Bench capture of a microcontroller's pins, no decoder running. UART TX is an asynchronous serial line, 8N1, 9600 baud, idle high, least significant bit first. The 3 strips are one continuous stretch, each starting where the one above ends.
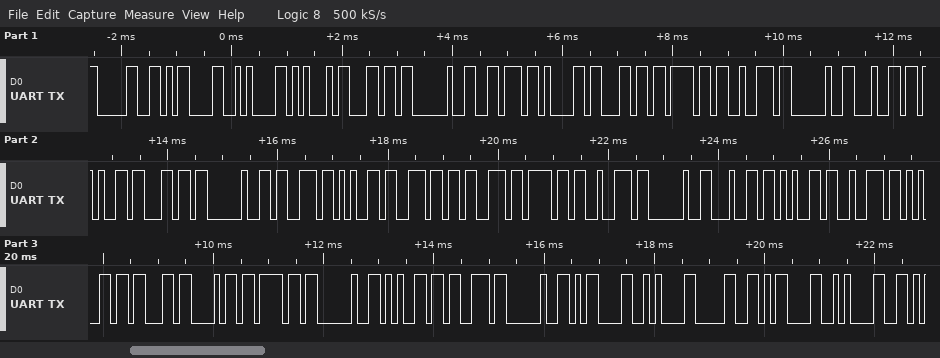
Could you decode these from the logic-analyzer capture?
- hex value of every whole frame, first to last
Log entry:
30 0D 0A 45 6C 20 76 61 6C 6F 72 20 64 65 6C 20 73 65 6E 73 6F 72 20 64 65 72 65 63 68 6F 20 65 73 20 0D 0A 30 0D 0A
